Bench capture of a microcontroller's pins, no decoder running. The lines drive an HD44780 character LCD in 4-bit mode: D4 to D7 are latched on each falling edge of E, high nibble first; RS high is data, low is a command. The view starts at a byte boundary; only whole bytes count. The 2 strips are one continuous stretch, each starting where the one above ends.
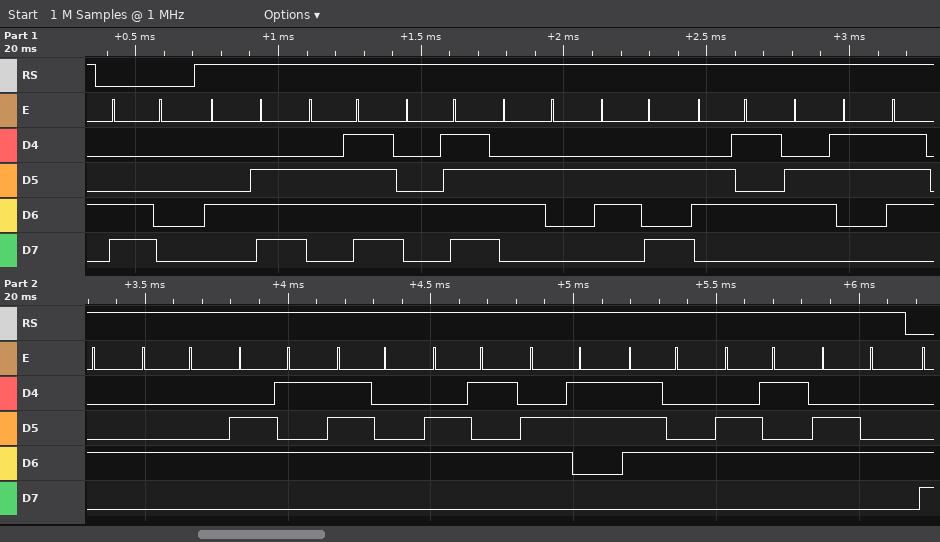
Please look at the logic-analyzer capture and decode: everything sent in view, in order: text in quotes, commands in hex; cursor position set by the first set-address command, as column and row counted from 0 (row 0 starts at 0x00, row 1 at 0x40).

0xC0 "NoObjectDetected"
column 0, row 1
